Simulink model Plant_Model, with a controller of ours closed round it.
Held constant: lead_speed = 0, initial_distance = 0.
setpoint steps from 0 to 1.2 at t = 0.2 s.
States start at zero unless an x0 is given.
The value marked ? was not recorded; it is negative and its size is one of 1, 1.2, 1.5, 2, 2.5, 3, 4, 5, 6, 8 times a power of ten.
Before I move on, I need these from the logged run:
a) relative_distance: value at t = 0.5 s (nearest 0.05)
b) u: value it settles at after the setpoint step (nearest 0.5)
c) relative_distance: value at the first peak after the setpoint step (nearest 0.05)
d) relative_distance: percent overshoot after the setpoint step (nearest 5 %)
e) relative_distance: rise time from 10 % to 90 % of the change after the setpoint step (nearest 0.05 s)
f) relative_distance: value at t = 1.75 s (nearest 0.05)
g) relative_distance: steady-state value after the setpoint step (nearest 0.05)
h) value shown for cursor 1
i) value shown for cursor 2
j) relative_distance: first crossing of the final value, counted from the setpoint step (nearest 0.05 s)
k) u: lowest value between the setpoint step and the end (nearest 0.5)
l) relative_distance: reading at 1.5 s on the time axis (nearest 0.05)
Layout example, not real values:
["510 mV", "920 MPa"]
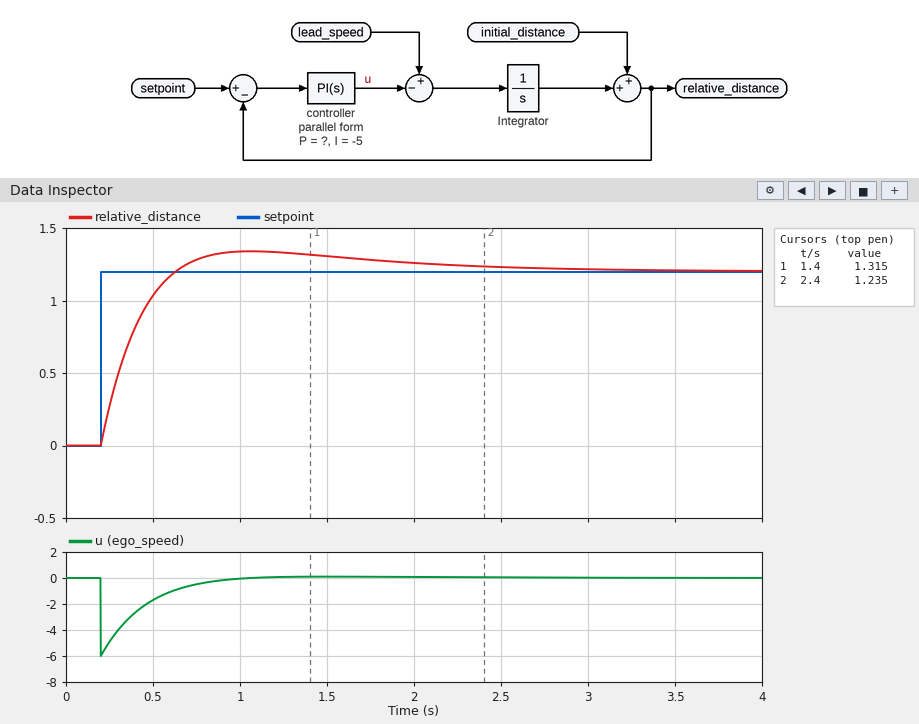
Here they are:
["1.05", "0.0", "1.35", "10 %", "0.30 s", "1.30", "1.20", "1.315", "1.235", "0.45 s", "-6.0", "1.30"]
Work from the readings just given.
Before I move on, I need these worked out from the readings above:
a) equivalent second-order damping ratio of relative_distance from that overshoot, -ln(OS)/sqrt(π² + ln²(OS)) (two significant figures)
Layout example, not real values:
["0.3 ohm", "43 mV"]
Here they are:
["0.59"]
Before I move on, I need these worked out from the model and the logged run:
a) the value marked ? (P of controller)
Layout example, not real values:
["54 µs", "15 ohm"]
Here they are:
["-5"]
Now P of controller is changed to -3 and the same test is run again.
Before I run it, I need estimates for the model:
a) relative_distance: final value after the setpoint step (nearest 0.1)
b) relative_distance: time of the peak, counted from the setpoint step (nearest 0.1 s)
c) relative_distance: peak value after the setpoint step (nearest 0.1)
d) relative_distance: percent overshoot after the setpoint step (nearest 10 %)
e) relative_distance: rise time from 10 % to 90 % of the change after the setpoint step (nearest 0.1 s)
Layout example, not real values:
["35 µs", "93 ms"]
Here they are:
["1.2", "1.0 s", "1.5", "20 %", "0.4 s"]
